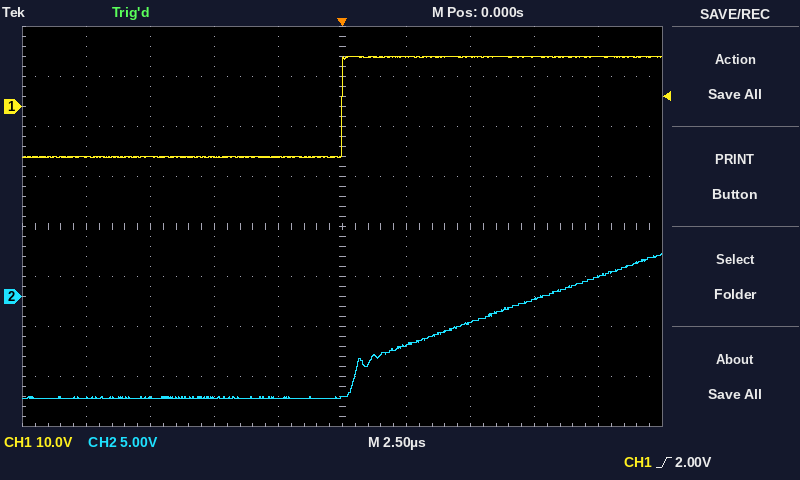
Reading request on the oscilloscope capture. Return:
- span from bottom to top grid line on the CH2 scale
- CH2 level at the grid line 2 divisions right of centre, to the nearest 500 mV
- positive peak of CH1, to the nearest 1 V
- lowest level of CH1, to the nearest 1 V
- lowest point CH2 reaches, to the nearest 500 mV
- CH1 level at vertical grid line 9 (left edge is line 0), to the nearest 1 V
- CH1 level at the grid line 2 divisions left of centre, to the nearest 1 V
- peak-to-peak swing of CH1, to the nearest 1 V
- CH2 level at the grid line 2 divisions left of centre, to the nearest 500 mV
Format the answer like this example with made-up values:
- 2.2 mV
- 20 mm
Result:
- 40 V
- -2.5 V
- 10 V
- -10 V
- -10.0 V
- 10 V
- -10 V
- 20 V
- -10.0 V
